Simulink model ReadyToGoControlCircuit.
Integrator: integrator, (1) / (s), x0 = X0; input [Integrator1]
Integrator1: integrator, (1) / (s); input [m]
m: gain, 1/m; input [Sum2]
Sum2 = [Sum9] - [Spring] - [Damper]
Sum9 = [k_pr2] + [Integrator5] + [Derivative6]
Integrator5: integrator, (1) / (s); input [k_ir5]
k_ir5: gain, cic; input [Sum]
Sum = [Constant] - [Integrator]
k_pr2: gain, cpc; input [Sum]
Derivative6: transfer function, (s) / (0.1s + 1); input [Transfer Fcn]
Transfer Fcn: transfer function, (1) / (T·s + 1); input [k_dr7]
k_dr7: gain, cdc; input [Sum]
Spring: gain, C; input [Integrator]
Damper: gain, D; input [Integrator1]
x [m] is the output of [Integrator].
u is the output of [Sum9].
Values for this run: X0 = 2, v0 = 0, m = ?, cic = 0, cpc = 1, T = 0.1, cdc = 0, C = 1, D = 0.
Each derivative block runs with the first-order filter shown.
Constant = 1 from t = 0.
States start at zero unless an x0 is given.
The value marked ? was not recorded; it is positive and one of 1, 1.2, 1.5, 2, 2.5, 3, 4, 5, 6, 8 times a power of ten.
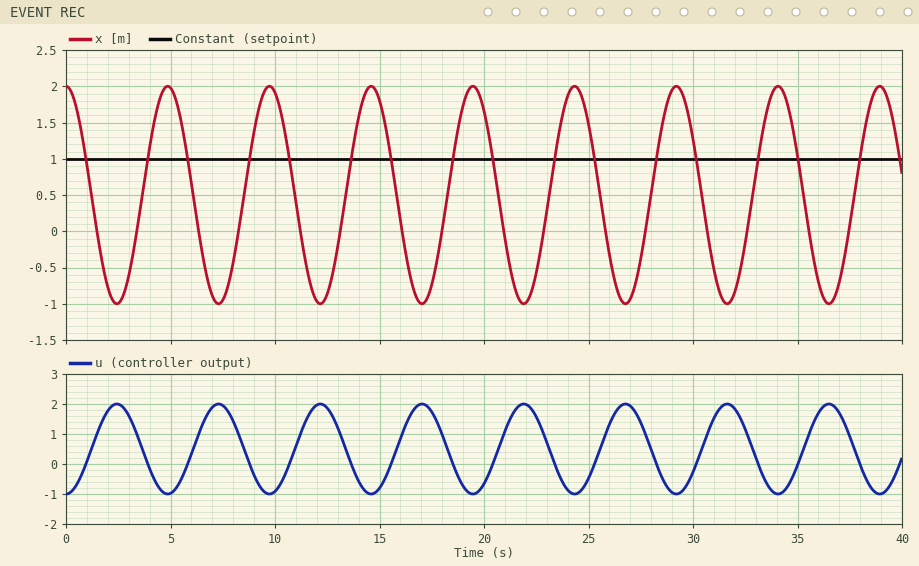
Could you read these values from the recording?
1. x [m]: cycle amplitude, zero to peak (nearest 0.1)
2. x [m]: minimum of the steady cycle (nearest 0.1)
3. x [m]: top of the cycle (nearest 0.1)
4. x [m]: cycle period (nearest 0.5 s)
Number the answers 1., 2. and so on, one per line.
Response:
1. 1.5
2. -1.0
3. 2.0
4. 5.0 s
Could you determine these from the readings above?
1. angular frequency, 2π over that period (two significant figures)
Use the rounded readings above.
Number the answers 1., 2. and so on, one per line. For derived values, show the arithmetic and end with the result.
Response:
1. 2π / 5 = 1.3 rad/s
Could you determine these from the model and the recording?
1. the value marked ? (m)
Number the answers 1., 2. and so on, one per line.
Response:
1. 1.2
